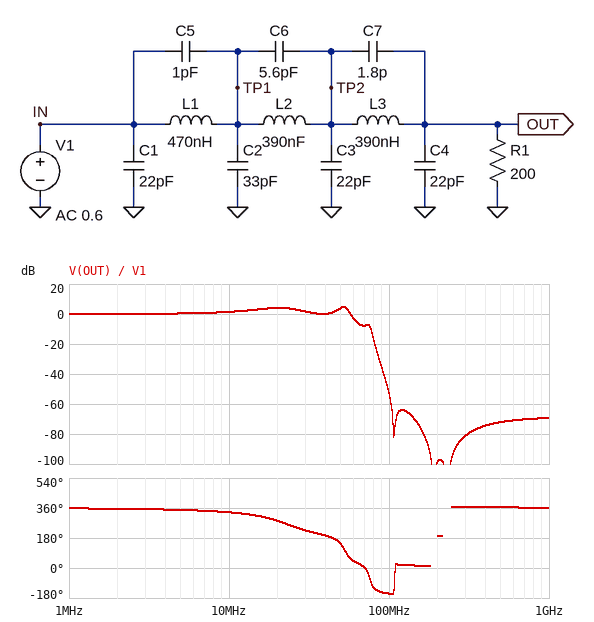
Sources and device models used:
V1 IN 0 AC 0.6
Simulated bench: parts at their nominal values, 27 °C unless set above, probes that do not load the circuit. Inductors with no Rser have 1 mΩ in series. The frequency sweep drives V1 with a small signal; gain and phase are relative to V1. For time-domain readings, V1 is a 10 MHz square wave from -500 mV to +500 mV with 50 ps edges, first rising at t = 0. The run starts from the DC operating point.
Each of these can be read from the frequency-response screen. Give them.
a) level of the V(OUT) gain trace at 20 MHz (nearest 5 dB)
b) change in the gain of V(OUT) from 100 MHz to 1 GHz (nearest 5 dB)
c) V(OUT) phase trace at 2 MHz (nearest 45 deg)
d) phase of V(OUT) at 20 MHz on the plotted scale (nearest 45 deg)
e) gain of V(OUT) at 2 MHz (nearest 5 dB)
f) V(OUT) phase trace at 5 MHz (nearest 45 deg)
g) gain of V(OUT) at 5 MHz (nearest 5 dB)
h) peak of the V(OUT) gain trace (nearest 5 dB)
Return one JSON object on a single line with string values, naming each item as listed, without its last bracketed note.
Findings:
{"level of the V(OUT) gain trace at 20 MHz": "5 dB", "change in the gain of V(OUT) from 100 MHz to 1 GHz": "-15 dB", "V(OUT) phase trace at 2 MHz": "360 deg", "phase of V(OUT) at 20 MHz on the plotted scale": "270 deg", "gain of V(OUT) at 2 MHz": "0 dB", "V(OUT) phase trace at 5 MHz": "360 deg", "gain of V(OUT) at 5 MHz": "0 dB", "peak of the V(OUT) gain trace": "5 dB"}
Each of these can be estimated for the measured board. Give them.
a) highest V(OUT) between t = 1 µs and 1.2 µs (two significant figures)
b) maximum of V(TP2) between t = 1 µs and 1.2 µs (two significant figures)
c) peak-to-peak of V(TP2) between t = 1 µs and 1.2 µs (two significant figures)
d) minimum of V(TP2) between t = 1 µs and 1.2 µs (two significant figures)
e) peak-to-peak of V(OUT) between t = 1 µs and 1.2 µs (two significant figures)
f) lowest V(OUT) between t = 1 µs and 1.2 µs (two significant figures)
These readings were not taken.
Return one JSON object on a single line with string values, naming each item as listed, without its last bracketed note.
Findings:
{"highest V(OUT) between t = 1 µs and 1.2 µs": "950 mV", "maximum of V(TP2) between t = 1 µs and 1.2 µs": "730 mV", "peak-to-peak of V(TP2) between t = 1 µs and 1.2 µs": "1.5 V", "minimum of V(TP2) between t = 1 µs and 1.2 µs": "-730 mV", "peak-to-peak of V(OUT) between t = 1 µs and 1.2 µs": "1.9 V", "lowest V(OUT) between t = 1 µs and 1.2 µs": "-950 mV"}
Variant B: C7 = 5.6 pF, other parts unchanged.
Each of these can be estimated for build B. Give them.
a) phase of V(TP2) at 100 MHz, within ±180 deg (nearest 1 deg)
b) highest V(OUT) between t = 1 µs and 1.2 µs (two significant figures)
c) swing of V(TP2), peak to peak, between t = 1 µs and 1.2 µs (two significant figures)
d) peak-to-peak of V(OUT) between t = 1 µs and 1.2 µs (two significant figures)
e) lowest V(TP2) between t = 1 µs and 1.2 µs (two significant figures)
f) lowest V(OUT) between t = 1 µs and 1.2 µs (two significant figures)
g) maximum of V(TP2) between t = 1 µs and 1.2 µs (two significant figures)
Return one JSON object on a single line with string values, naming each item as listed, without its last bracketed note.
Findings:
{"phase of V(TP2) at 100 MHz, within ±180 deg": "0 deg", "highest V(OUT) between t = 1 µs and 1.2 µs": "1.1 V", "swing of V(TP2), peak to peak, between t = 1 µs and 1.2 µs": "1.9 V", "peak-to-peak of V(OUT) between t = 1 µs and 1.2 µs": "2.1 V", "lowest V(TP2) between t = 1 µs and 1.2 µs": "-950 mV", "lowest V(OUT) between t = 1 µs and 1.2 µs": "-1.1 V", "maximum of V(TP2) between t = 1 µs and 1.2 µs": "950 mV"}
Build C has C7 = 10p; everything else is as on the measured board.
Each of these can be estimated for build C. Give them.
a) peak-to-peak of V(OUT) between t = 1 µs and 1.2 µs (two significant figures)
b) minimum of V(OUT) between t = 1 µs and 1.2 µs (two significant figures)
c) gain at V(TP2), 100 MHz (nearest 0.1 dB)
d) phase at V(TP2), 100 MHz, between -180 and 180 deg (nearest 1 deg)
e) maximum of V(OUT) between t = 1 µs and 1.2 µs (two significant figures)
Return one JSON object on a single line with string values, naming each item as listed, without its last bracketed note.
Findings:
{"peak-to-peak of V(OUT) between t = 1 µs and 1.2 µs": "2.0 V", "minimum of V(OUT) between t = 1 µs and 1.2 µs": "-1.0 V", "gain at V(TP2), 100 MHz": "-44.6 dB", "phase at V(TP2), 100 MHz, between -180 and 180 deg": "0 deg", "maximum of V(OUT) between t = 1 µs and 1.2 µs": "1.0 V"}
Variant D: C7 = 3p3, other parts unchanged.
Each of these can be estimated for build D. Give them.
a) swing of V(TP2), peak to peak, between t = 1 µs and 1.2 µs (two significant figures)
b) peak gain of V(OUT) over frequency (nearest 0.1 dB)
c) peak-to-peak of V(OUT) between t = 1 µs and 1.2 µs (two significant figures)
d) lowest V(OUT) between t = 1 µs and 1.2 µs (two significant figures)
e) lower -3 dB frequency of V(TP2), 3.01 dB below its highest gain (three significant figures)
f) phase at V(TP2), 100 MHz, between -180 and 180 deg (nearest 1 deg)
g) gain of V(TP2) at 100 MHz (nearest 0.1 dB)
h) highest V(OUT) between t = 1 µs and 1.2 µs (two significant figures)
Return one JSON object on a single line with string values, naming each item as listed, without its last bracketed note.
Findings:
{"swing of V(TP2), peak to peak, between t = 1 µs and 1.2 µs": "1.5 V", "peak gain of V(OUT) over frequency": "4.6 dB", "peak-to-peak of V(OUT) between t = 1 µs and 1.2 µs": "2.0 V", "lowest V(OUT) between t = 1 µs and 1.2 µs": "-980 mV", "lower -3 dB frequency of V(TP2), 3.01 dB below its highest gain": "3.05 MHz", "phase at V(TP2), 100 MHz, between -180 and 180 deg": "1 deg", "gain of V(TP2) at 100 MHz": "-41.8 dB", "highest V(OUT) between t = 1 µs and 1.2 µs": "980 mV"}
